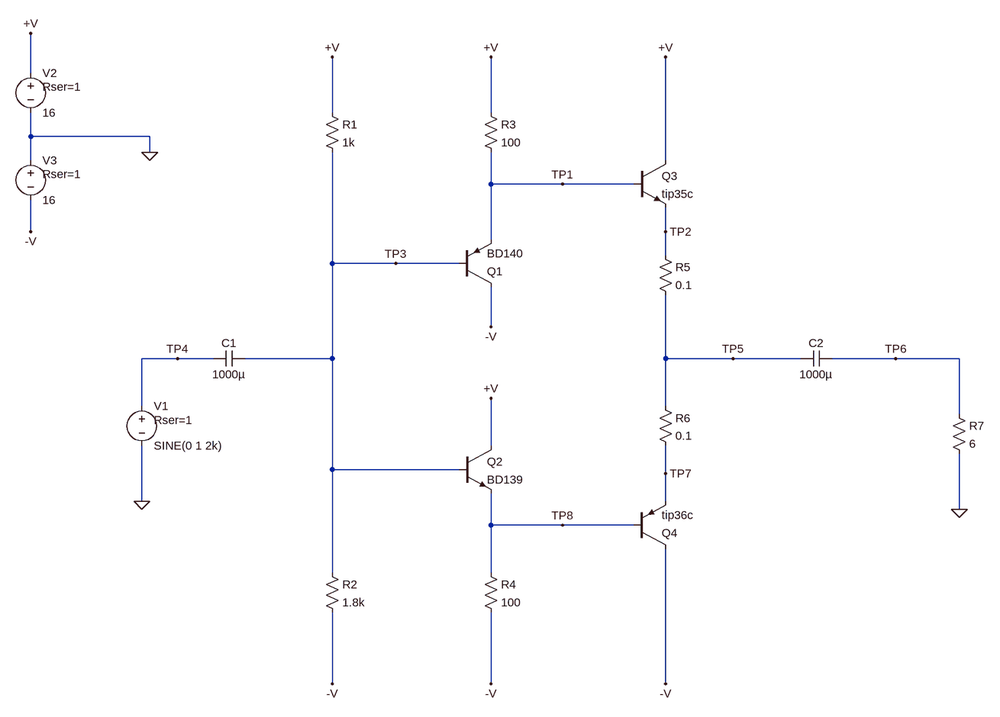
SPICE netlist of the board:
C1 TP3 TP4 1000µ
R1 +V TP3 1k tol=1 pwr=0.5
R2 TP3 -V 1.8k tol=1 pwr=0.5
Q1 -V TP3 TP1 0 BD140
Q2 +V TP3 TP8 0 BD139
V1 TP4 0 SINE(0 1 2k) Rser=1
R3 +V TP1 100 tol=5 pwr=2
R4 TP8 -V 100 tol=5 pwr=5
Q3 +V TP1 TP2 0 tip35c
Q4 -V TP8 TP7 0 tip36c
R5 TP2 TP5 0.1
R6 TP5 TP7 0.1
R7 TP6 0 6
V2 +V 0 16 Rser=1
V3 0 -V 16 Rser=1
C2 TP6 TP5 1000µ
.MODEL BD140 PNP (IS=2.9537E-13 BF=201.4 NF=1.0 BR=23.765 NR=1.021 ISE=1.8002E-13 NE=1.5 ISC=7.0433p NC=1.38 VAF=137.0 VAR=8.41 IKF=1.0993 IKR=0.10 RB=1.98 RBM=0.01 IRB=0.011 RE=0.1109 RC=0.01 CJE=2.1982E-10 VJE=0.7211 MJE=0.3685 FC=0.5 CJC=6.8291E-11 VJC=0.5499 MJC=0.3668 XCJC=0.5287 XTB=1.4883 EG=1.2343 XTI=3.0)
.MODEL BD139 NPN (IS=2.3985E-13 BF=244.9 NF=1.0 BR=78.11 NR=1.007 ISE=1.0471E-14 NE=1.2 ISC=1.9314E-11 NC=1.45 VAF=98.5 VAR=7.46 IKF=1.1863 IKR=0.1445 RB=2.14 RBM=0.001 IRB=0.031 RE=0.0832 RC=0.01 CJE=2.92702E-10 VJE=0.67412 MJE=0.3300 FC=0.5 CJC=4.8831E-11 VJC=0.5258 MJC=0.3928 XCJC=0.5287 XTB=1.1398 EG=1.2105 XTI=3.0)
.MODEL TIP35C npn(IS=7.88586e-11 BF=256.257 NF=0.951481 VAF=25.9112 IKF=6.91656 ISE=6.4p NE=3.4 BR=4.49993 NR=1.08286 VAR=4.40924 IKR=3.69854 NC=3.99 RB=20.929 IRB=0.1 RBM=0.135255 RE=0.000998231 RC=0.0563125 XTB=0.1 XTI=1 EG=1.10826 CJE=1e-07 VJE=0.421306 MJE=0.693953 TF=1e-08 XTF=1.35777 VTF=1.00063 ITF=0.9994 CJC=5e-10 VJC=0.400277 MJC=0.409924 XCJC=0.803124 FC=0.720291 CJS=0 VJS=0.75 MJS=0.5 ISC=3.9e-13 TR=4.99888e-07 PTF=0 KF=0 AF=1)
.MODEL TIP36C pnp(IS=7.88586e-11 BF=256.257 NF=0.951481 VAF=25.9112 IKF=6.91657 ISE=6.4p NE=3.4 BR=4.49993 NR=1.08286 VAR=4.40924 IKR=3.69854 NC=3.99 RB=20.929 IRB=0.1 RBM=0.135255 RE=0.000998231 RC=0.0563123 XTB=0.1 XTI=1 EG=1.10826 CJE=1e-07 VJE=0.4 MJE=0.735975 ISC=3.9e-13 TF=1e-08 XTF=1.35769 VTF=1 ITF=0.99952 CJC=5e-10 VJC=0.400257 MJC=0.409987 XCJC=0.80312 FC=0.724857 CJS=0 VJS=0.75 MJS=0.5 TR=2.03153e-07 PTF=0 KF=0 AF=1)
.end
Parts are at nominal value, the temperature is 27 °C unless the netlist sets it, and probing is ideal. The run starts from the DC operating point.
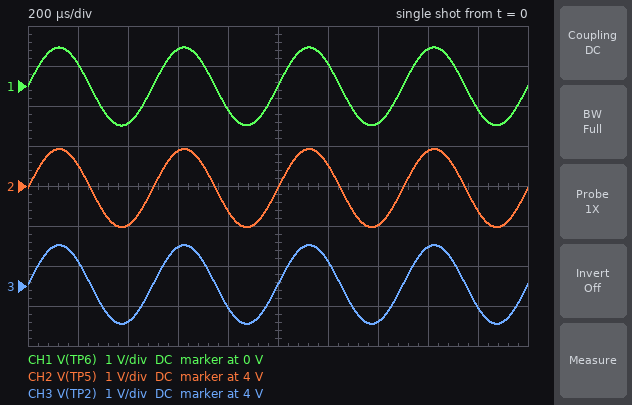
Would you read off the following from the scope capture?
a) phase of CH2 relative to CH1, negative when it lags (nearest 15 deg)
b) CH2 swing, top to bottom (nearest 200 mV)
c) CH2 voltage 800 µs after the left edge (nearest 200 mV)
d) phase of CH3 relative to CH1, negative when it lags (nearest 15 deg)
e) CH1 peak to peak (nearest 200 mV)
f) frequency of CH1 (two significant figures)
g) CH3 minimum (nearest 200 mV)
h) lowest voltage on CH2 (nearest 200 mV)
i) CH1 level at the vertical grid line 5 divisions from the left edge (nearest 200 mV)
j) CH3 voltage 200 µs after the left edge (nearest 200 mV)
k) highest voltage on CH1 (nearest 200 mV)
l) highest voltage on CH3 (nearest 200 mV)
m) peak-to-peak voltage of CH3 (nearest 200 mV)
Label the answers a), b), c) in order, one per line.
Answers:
a) 0 deg
b) 2.0 V
c) 3.4 V
d) 0 deg
e) 2.0 V
f) 2.0 kHz
g) 3.0 V
h) 3.0 V
i) 0 V
j) 4.6 V
k) 1.0 V
l) 5.0 V
m) 2.0 V
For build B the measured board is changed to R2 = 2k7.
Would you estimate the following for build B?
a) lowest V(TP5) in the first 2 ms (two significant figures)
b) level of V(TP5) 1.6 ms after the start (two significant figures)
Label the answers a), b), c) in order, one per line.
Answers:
a) 5.3 V
b) 7.2 V
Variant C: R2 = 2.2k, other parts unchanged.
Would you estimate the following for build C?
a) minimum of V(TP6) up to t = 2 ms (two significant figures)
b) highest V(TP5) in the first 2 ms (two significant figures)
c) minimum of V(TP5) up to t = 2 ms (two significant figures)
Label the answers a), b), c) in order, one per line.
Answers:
a) -990 mV
b) 6.1 V
c) 4.2 V
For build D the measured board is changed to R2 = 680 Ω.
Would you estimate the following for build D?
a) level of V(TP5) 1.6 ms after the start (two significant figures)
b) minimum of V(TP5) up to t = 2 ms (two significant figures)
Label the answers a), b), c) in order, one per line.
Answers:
a) -1.7 V
b) -3.6 V
